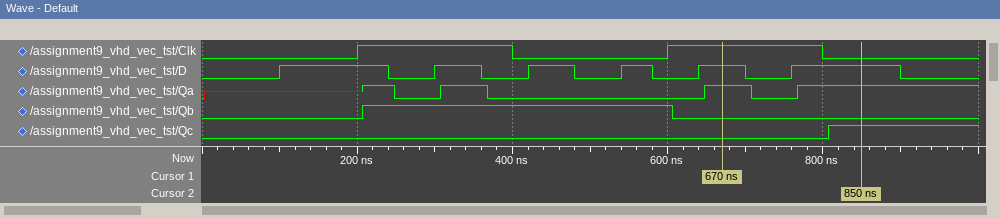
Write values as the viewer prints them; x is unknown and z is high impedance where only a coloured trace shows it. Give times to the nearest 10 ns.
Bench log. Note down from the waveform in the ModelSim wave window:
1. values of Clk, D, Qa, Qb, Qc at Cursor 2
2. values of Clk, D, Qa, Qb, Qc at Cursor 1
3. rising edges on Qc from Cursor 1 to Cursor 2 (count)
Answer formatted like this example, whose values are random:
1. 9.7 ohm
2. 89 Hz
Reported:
1. Clk=0, D=1, Qa=1, Qb=0, Qc=1
2. Clk=1, D=1, Qa=1, Qb=0, Qc=0
3. 1
